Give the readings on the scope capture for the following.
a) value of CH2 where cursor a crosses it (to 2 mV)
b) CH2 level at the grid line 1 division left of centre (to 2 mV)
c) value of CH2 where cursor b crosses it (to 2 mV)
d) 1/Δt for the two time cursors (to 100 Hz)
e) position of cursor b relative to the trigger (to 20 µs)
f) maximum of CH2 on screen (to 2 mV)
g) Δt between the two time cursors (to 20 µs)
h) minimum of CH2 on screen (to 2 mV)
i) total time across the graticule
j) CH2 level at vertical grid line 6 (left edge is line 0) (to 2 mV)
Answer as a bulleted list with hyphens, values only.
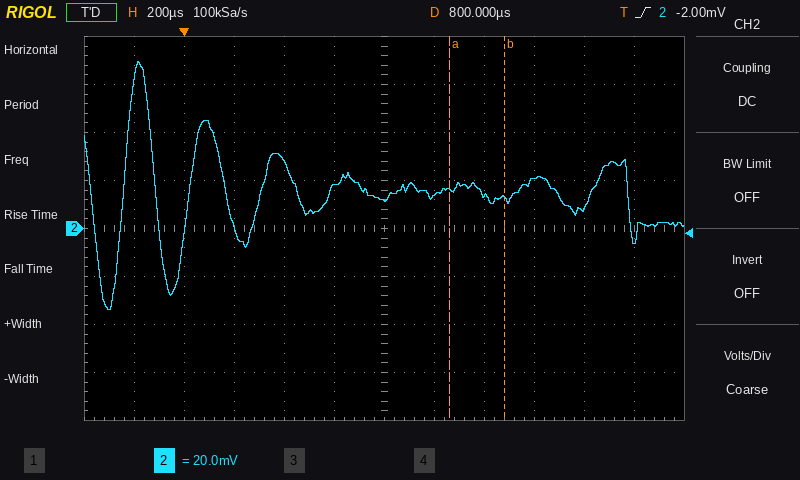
- 16 mV
- 18 mV
- 12 mV
- 4.5 kHz
- +1.28 ms
- 70 mV
- 220 µs
- -34 mV
- 2.4 ms
- 12 mV
